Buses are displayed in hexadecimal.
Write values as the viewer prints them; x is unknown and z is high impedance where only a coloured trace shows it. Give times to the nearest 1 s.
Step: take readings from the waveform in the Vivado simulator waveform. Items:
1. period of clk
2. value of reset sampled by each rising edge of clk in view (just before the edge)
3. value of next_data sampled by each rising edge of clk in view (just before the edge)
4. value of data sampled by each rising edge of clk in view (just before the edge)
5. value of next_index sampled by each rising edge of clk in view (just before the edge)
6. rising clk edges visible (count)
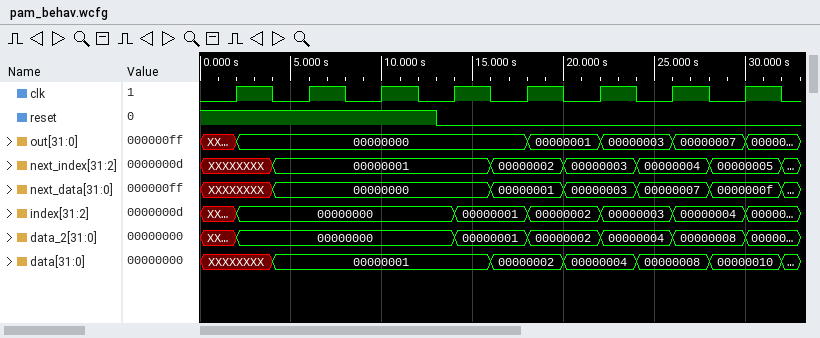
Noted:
4 s
1 1 1 0 0 0 0 0
XXXXXXXX, 00000000, 00000000, 00000000, 00000001, 00000003, 00000007, 0000000f
XXXXXXXX, 00000001, 00000001, 00000001, 00000002, 00000004, 00000008, 00000010
XXXXXXXX, 00000001, 00000001, 00000001, 00000002, 00000003, 00000004, 00000005
8
